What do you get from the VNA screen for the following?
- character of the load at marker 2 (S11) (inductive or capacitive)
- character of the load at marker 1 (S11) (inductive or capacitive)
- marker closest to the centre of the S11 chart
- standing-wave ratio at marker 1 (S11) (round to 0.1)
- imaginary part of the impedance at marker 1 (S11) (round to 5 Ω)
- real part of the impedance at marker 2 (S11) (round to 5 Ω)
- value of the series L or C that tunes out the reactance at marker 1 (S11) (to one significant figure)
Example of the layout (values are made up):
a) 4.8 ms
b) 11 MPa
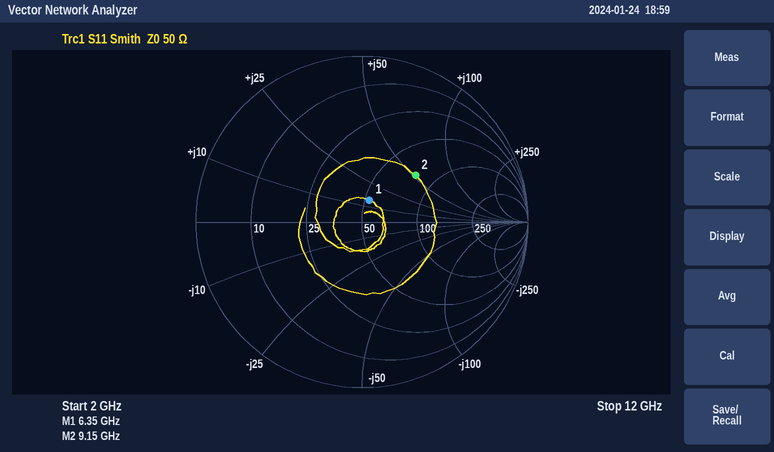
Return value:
a) inductive
b) inductive
c) marker 1
d) 1.3
e) +15 Ω
f) 75 Ω
g) 2 pF
